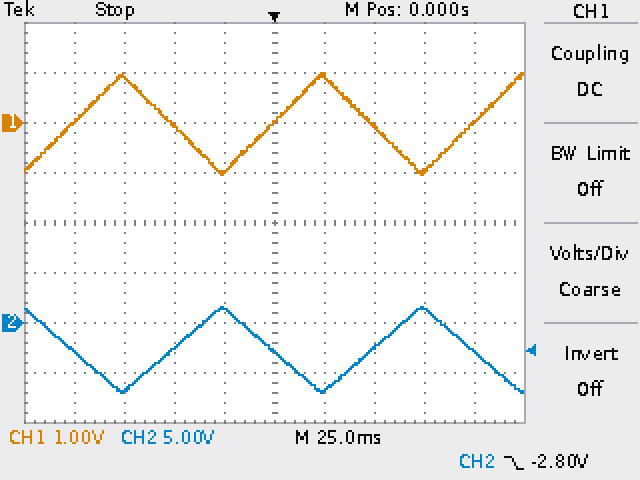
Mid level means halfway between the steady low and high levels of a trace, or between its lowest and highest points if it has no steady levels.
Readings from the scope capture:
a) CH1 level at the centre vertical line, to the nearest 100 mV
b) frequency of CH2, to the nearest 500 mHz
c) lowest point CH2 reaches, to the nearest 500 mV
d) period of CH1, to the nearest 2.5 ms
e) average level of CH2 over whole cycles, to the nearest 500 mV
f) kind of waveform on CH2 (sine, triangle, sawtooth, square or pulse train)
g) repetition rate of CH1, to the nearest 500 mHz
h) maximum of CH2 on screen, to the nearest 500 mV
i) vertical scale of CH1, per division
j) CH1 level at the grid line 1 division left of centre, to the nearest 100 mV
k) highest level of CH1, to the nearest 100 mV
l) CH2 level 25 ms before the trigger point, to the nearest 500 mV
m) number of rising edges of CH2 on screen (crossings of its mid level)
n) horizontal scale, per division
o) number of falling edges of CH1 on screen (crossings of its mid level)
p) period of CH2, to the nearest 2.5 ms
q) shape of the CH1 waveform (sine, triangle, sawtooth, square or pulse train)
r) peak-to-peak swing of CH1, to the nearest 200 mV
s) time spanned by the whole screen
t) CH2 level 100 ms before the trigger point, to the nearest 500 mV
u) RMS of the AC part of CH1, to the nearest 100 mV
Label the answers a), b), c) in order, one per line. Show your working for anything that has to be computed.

a) 0.0 V
b) 1 / 100.0 ms ≈ 10.0 Hz
c) -7.0 V
d) 100.0 ms
e) (1.5 V + (-7.0 V)) / 2 ≈ -2.75 V, so -2.5 V to the nearest 500 mV
f) triangle
g) 1 / 100.0 ms ≈ 10.0 Hz
h) 1.5 V
i) 1 V
j) -1.0 V
k) 1.0 V
l) 1.5 V
m) 2
n) 25 ms
o) 2
p) 100.0 ms
q) triangle
r) 2.0 V
s) 250 ms
t) -3.0 V
u) 2.0 V / (2√3) ≈ 577 mV, so 600 mV to the nearest 100 mV
